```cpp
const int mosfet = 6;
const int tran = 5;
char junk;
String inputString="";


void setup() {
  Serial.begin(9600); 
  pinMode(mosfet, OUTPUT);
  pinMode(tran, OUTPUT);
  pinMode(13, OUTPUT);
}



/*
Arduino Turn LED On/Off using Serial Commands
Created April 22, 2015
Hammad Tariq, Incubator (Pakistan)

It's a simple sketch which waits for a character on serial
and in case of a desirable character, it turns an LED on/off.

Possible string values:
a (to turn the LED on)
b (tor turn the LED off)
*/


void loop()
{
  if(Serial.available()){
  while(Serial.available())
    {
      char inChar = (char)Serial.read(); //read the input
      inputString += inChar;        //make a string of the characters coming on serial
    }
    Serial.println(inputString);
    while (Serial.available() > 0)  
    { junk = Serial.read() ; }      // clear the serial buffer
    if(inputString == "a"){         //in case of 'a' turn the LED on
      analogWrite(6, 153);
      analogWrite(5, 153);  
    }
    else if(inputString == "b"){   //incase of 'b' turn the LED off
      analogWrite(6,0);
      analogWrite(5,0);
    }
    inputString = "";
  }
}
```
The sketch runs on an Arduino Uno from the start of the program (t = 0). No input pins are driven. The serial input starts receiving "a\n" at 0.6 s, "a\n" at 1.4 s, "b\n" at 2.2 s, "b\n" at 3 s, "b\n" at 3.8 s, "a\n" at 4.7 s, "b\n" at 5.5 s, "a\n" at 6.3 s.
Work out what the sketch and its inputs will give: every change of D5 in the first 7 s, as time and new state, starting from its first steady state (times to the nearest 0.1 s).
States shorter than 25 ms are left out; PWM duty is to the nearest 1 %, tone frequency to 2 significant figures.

0 s low; 0.6 s PWM 60 %; 2.2 s low; 4.7 s PWM 60 %; 5.5 s low; 6.3 s PWM 60 %
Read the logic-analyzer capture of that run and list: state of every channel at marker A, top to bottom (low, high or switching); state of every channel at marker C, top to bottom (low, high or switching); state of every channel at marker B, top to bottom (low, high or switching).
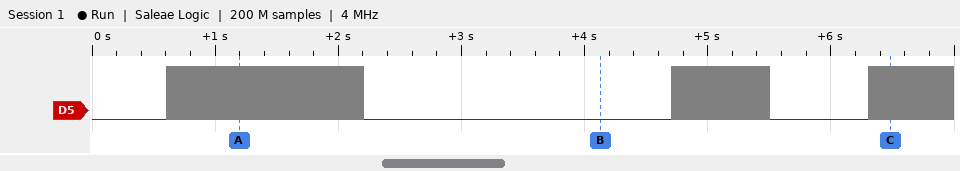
D5 switching
D5 switching
D5 low
